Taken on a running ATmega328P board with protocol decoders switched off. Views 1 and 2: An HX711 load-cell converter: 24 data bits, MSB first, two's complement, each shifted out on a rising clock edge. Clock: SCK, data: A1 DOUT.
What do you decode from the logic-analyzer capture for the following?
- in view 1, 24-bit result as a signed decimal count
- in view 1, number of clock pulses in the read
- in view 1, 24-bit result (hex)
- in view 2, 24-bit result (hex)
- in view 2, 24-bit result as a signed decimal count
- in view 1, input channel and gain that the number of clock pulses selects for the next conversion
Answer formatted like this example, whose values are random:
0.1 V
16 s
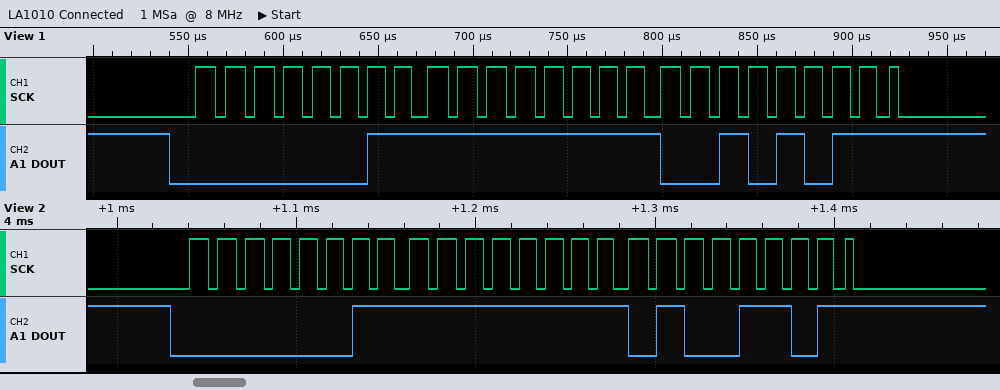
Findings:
261931
25
0x03FF2B
0x03FF4D
261965
channel A, gain 128
